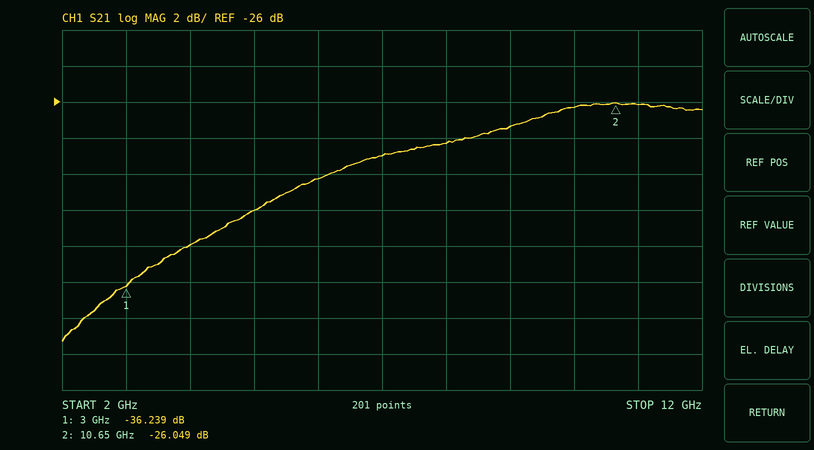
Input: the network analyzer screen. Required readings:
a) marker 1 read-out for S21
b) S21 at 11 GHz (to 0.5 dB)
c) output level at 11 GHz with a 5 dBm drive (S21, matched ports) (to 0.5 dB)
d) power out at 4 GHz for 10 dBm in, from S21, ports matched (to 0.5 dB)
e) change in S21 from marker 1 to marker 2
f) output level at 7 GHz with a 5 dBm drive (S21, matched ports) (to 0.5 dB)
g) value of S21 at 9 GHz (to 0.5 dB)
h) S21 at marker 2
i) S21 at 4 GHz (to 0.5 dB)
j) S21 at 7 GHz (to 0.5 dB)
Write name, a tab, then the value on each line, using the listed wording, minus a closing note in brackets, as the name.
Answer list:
marker 1 read-out for S21	-36.239 dB
S21 at 11 GHz	-26.0 dB
output level at 11 GHz with a 5 dBm drive (S21, matched ports)	-21.0 dBm
power out at 4 GHz for 10 dBm in, from S21, ports matched	-24.0 dBm
change in S21 from marker 1 to marker 2	10.190 dB
output level at 7 GHz with a 5 dBm drive (S21, matched ports)	-24.0 dBm
value of S21 at 9 GHz	-27.5 dB
S21 at marker 2	-26.049 dB
S21 at 4 GHz	-34.0 dB
S21 at 7 GHz	-29.0 dB
